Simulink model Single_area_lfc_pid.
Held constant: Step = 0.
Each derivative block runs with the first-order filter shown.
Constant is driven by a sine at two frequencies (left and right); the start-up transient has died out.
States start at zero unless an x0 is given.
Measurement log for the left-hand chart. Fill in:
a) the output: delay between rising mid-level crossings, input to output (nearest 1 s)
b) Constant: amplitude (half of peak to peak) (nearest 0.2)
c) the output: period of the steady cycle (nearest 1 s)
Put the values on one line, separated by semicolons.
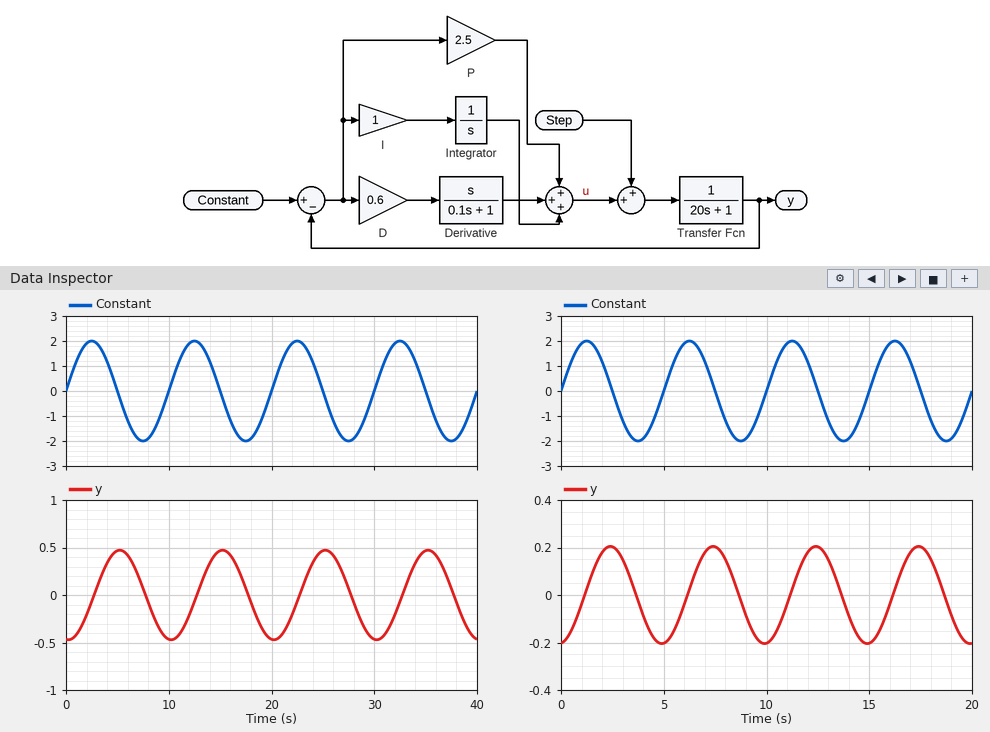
3 s; 2.0; 10 s
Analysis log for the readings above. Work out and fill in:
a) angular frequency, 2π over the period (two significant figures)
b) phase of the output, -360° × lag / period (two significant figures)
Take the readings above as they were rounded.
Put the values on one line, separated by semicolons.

0.63 rad/s; -110°
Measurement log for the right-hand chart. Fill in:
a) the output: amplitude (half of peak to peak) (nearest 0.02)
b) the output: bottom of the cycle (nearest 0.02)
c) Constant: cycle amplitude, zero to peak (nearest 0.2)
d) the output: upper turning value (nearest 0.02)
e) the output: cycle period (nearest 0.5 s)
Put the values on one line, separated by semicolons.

0.20; -0.20; 2.0; 0.20; 5.0 s
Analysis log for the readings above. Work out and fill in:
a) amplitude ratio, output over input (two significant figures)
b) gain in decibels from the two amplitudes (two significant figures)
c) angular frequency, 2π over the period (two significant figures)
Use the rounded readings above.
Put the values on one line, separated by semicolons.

0.10; -20 dB; 1.3 rad/s
